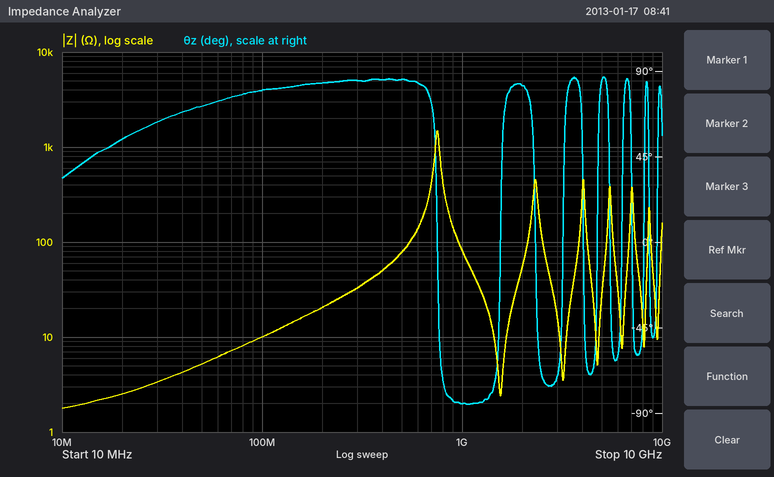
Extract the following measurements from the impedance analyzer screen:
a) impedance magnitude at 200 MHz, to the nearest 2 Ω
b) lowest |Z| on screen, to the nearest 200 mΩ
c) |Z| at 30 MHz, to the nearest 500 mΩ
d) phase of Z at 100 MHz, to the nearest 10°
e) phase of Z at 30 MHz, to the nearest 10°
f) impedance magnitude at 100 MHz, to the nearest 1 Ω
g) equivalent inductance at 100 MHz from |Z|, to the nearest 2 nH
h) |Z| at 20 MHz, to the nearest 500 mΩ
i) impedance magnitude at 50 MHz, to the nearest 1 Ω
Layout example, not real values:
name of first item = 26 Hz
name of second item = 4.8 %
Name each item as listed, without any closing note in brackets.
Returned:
impedance magnitude at 200 MHz, to the nearest 2 Ω = 20 Ω
lowest |Z| on screen, to the nearest 200 mΩ = 1.8 Ω
|Z| at 30 MHz, to the nearest 500 mΩ = 3.5 Ω
phase of Z at 100 MHz, to the nearest 10° = 80°
phase of Z at 30 MHz, to the nearest 10° = 60°
impedance magnitude at 100 MHz, to the nearest 1 Ω = 10 Ω
equivalent inductance at 100 MHz from |Z|, to the nearest 2 nH = 16 nH
|Z| at 20 MHz, to the nearest 500 mΩ = 2.5 Ω
impedance magnitude at 50 MHz, to the nearest 1 Ω = 5 Ω
